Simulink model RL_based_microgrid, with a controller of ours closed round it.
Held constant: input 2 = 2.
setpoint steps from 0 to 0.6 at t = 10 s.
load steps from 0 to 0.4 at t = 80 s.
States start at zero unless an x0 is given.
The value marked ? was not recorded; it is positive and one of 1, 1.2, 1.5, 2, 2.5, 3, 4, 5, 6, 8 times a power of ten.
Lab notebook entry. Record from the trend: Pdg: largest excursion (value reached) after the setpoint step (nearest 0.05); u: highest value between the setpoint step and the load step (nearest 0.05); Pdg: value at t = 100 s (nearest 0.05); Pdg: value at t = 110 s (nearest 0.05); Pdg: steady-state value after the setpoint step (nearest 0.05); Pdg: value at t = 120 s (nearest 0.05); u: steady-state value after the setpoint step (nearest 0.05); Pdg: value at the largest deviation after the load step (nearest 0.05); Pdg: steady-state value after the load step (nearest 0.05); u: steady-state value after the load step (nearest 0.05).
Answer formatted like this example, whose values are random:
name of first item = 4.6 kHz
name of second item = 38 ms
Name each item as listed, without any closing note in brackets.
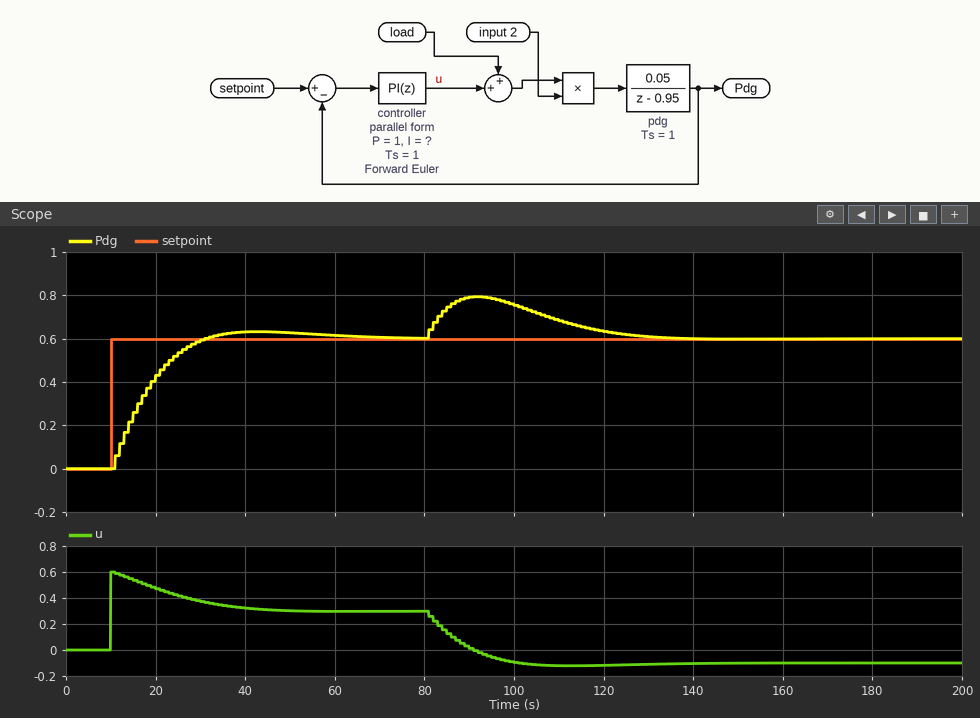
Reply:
Pdg: largest excursion (value reached) after the setpoint step = 0.65
u: highest value between the setpoint step and the load step = 0.60
Pdg: value at t = 100 s = 0.75
Pdg: value at t = 110 s = 0.70
Pdg: steady-state value after the setpoint step = 0.60
Pdg: value at t = 120 s = 0.65
u: steady-state value after the setpoint step = 0.30
Pdg: value at the largest deviation after the load step = 0.80
Pdg: steady-state value after the load step = 0.60
u: steady-state value after the load step = -0.10
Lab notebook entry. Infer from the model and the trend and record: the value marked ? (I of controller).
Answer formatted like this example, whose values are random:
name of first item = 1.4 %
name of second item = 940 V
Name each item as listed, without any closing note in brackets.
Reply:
the value marked ? = 0.08
